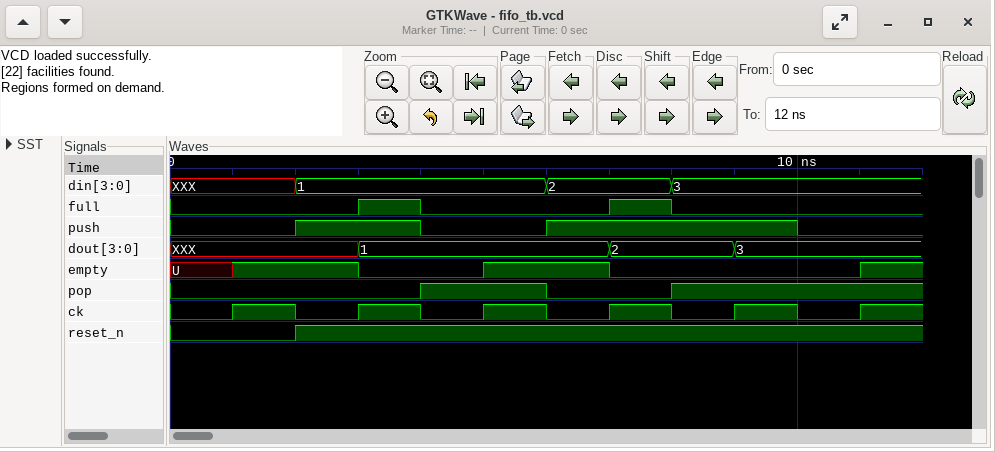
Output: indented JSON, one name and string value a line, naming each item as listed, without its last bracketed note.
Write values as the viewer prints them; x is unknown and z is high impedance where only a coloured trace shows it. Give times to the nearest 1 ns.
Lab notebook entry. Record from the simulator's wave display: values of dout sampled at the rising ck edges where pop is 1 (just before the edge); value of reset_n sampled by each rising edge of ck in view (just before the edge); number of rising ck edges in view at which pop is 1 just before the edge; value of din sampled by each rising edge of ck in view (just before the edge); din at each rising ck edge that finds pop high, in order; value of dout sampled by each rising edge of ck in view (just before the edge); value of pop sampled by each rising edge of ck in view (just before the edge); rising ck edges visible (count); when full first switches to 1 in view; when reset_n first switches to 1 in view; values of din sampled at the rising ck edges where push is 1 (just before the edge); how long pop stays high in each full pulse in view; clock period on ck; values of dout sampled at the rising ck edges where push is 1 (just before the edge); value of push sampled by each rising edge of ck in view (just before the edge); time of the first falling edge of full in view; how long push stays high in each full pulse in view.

{
  "values of dout sampled at the rising ck edges where pop is 1": "1, 2, 3",
  "value of reset_n sampled by each rising edge of ck in view": "0 1 1 1 1 1",
  "number of rising ck edges in view at which pop is 1 just before the edge": "3",
  "value of din sampled by each rising edge of ck in view": "XXX, 1, 1, 2, 3, 3",
  "din at each rising ck edge that finds pop high, in order": "1, 3, 3",
  "value of dout sampled by each rising edge of ck in view": "XXX, XXX, 1, 1, 2, 3",
  "value of pop sampled by each rising edge of ck in view": "0 0 1 0 1 1",
  "rising ck edges visible": "6",
  "when full first switches to 1 in view": "3 ns",
  "when reset_n first switches to 1 in view": "2 ns",
  "values of din sampled at the rising ck edges where push is 1": "1, 2, 3",
  "how long pop stays high in each full pulse in view": "2 ns",
  "clock period on ck": "2 ns",
  "values of dout sampled at the rising ck edges where push is 1": "XXX, 1, 2",
  "value of push sampled by each rising edge of ck in view": "0 1 0 1 1 0",
  "time of the first falling edge of full in view": "4 ns",
  "how long push stays high in each full pulse in view": "2 ns, 4 ns"
}
